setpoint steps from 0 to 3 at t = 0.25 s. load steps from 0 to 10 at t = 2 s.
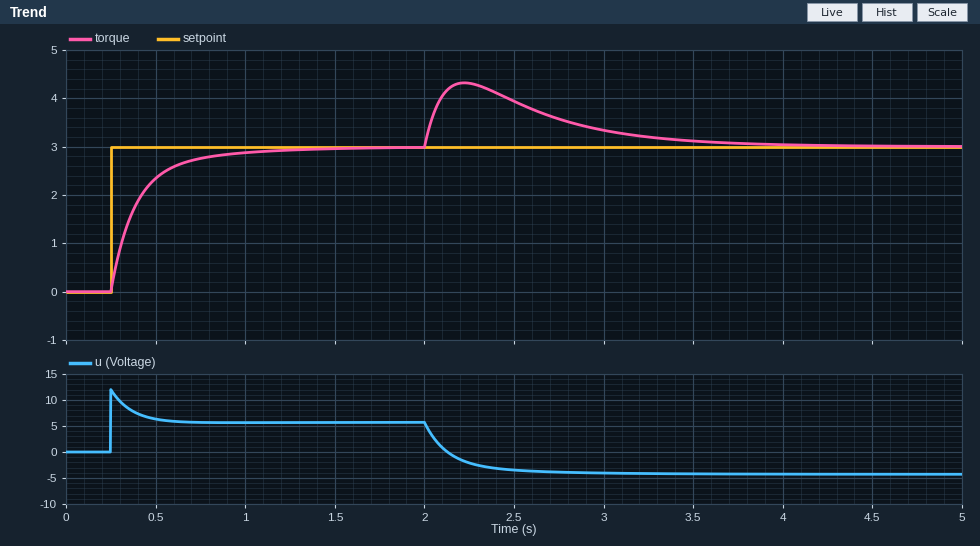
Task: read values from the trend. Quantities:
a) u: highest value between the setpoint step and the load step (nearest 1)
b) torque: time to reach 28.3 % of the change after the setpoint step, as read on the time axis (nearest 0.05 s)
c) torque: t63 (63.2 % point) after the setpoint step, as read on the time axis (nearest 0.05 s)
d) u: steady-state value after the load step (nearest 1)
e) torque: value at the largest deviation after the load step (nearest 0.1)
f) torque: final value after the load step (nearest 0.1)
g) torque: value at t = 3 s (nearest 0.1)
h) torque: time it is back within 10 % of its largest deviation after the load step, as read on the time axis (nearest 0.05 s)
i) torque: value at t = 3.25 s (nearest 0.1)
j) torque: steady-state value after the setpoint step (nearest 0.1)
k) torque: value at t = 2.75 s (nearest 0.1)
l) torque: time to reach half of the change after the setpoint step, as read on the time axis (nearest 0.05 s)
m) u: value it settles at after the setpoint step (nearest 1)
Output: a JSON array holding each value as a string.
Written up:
["12", "0.30 s", "0.40 s", "-4", "4.3", "3.0", "3.3", "3.45 s", "3.2", "3.0", "3.6", "0.35 s", "6"]
